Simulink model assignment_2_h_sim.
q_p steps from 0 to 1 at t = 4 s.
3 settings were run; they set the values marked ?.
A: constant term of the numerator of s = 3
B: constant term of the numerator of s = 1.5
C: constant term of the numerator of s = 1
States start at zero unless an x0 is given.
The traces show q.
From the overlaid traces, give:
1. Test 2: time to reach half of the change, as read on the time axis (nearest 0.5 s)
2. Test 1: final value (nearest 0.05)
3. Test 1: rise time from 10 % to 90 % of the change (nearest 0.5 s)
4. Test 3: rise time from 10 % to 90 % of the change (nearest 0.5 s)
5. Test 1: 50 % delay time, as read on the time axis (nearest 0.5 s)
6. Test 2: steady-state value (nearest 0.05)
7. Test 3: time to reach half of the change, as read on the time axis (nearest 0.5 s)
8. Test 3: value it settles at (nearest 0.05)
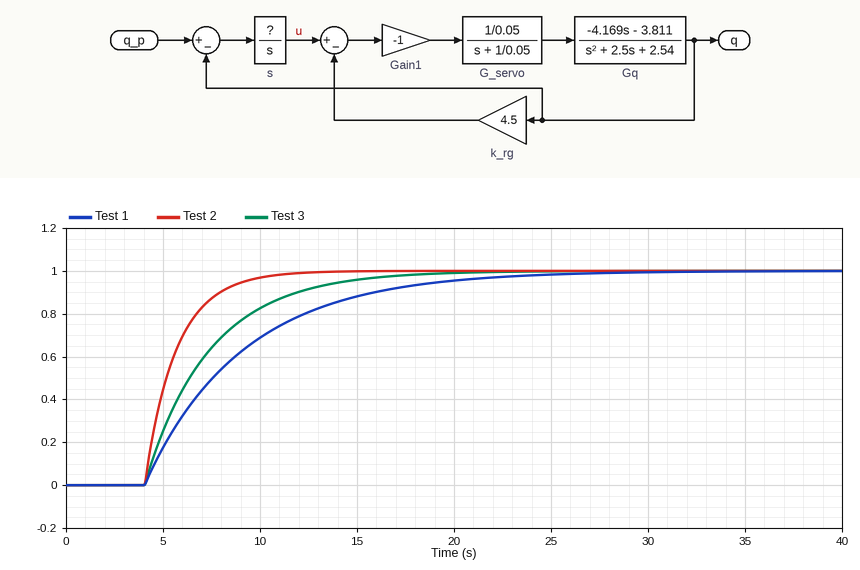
5.0 s
1.00
11.5 s
7.5 s
7.5 s
1.00
6.5 s
1.00
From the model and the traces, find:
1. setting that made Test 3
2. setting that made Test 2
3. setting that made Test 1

B
A
C
